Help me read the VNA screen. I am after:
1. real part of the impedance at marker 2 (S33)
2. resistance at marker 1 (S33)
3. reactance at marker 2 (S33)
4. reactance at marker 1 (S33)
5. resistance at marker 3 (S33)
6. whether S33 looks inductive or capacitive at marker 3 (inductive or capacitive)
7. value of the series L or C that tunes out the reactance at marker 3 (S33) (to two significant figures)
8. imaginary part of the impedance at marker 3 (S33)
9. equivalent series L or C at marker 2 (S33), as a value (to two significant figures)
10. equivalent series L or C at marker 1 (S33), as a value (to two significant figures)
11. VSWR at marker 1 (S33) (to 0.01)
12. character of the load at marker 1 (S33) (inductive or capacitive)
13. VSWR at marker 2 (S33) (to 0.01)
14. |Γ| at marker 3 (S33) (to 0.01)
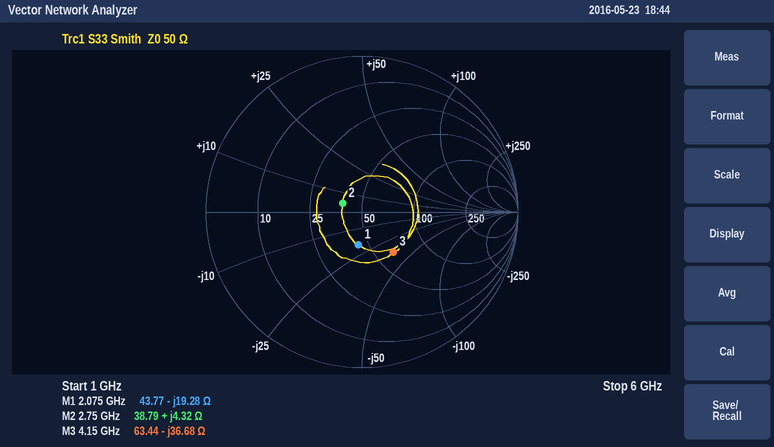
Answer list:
38.79 Ω
43.77 Ω
+4.32 Ω
-19.28 Ω
63.44 Ω
capacitive
1.4 nH
-36.68 Ω
250 pH
4.0 pF
1.54
capacitive
1.31
0.33
